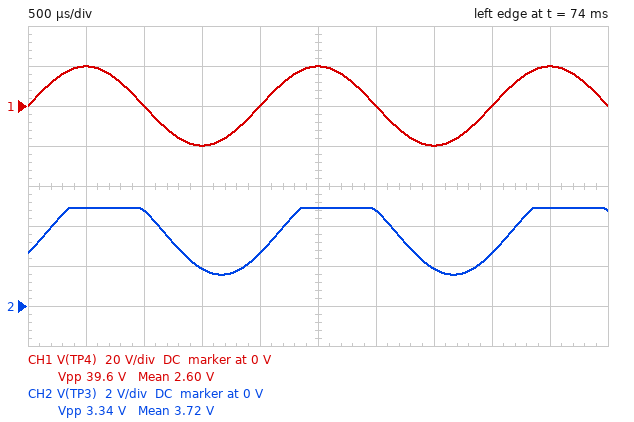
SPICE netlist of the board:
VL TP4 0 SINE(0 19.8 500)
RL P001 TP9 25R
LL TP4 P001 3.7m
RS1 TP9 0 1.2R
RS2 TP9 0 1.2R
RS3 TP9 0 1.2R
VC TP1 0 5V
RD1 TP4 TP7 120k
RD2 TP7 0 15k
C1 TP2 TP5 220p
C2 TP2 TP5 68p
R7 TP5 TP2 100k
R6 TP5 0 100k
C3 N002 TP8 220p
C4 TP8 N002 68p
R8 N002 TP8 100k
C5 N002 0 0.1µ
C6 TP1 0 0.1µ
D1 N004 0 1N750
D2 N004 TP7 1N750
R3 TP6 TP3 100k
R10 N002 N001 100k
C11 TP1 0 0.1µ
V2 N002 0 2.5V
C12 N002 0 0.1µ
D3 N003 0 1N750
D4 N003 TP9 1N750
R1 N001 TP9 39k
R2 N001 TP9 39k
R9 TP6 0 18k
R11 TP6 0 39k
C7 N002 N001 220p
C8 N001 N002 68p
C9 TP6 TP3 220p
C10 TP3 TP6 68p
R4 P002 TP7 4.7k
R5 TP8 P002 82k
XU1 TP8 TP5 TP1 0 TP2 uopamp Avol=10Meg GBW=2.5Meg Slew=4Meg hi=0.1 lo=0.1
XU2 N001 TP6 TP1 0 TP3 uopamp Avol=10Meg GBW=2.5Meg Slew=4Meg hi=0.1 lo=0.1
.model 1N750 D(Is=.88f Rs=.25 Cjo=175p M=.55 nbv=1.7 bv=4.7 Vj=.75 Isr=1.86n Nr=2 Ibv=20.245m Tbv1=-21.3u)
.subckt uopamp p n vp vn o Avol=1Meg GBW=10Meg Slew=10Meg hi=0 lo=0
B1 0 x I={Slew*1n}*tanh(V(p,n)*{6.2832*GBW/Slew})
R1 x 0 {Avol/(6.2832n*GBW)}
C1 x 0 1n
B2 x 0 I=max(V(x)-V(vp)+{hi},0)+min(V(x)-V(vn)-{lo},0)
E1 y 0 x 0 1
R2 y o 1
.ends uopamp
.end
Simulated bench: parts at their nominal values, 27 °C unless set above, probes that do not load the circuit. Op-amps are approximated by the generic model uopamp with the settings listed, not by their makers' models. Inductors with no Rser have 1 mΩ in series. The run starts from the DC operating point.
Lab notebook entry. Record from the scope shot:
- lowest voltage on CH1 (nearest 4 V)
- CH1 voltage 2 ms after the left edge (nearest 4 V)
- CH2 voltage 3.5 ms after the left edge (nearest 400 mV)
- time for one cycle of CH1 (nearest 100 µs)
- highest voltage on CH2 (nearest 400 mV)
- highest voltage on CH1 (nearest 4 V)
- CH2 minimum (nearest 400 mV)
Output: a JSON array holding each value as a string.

["-20 V", "0 V", "2.0 V", "2.0 ms", "4.8 V", "20 V", "1.6 V"]
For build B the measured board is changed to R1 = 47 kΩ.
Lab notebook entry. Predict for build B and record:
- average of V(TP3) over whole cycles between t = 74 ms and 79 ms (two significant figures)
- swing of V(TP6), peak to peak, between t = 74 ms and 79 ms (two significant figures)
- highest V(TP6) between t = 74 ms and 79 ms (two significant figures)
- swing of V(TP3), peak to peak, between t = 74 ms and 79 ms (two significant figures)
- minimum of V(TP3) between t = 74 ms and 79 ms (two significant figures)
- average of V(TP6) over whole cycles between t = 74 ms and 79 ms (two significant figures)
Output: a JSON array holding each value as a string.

["3.7 V", "350 mV", "550 mV", "3.0 V", "1.9 V", "410 mV"]
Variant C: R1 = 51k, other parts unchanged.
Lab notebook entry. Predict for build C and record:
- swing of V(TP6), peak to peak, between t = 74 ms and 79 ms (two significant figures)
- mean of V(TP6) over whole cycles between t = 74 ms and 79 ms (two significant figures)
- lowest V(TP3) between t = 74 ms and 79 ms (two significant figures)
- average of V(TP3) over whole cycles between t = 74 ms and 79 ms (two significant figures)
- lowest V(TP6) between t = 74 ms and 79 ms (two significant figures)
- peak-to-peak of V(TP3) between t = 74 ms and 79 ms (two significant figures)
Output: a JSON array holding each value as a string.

["330 mV", "420 mV", "2.0 V", "3.8 V", "220 mV", "2.9 V"]
